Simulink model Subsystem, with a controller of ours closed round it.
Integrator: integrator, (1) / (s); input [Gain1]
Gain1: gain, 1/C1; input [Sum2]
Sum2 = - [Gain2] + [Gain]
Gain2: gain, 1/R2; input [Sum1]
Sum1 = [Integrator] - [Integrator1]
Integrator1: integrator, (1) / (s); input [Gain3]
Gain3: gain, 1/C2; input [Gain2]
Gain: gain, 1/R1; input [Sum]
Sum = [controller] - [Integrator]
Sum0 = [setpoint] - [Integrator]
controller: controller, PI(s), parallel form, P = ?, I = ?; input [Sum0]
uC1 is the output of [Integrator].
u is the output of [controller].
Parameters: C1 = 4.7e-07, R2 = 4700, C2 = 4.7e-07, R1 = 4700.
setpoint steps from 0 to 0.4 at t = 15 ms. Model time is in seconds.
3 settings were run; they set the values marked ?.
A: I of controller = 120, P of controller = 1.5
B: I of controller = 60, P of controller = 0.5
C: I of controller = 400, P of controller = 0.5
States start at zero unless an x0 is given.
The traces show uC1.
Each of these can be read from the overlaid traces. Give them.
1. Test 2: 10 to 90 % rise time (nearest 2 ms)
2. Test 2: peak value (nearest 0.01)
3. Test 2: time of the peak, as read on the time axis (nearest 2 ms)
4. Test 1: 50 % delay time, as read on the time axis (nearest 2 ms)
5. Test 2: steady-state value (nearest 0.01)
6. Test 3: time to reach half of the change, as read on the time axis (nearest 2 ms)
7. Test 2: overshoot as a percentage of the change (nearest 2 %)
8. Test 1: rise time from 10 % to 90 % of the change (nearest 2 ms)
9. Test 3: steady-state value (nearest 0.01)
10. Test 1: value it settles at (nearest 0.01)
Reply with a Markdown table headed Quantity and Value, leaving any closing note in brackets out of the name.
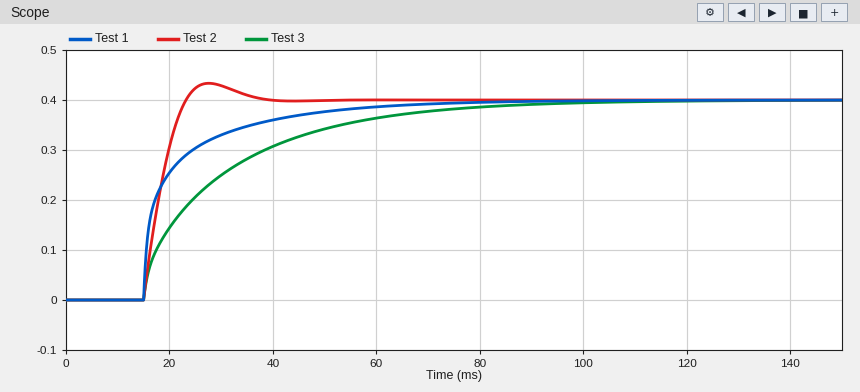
| Quantity | Value |
|---|---|
| Test 2: 10 to 90 % rise time | 6 ms |
| Test 2: peak value | 0.43 |
| Test 2: time of the peak, as read on the time axis | 28 ms |
| Test 1: 50 % delay time, as read on the time axis | 18 ms |
| Test 2: steady-state value | 0.40 |
| Test 3: time to reach half of the change, as read on the time axis | 24 ms |
| Test 2: overshoot as a percentage of the change | 8 % |
| Test 1: rise time from 10 % to 90 % of the change | 24 ms |
| Test 3: steady-state value | 0.40 |
| Test 1: value it settles at | 0.40 |
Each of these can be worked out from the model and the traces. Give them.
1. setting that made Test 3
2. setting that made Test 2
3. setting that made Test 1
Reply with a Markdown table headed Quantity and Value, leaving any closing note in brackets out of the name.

| Quantity | Value |
|---|---|
| setting that made Test 3 | B |
| setting that made Test 2 | C |
| setting that made Test 1 | A |
